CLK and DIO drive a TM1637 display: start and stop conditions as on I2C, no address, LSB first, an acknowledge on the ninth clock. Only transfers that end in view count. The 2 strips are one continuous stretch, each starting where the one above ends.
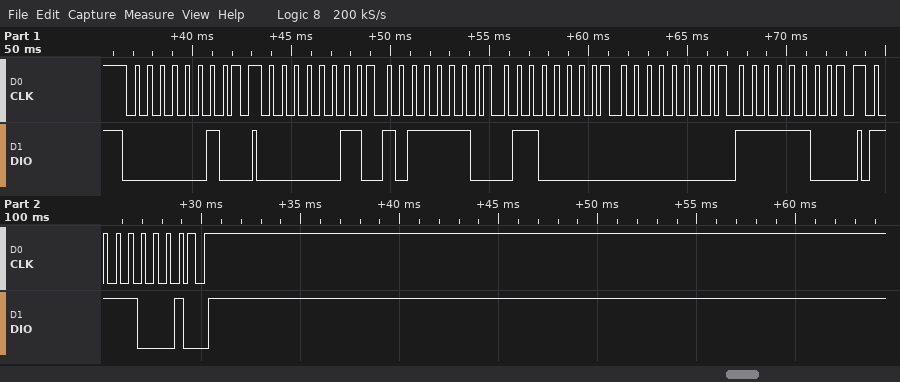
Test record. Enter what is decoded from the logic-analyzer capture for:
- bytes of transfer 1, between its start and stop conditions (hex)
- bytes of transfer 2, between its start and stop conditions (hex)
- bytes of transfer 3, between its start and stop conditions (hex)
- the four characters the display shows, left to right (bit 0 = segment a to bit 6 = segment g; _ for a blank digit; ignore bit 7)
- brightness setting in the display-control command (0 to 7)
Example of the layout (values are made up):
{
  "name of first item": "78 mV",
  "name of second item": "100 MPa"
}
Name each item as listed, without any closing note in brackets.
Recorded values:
{
  "bytes of transfer 1, between its start and stop conditions": "40",
  "bytes of transfer 2, between its start and stop conditions": "C0 7D 06 00 3F",
  "bytes of transfer 3, between its start and stop conditions": "8F",
  "the four characters the display shows, left to right": "61_0",
  "brightness setting in the display-control command": "7"
}
